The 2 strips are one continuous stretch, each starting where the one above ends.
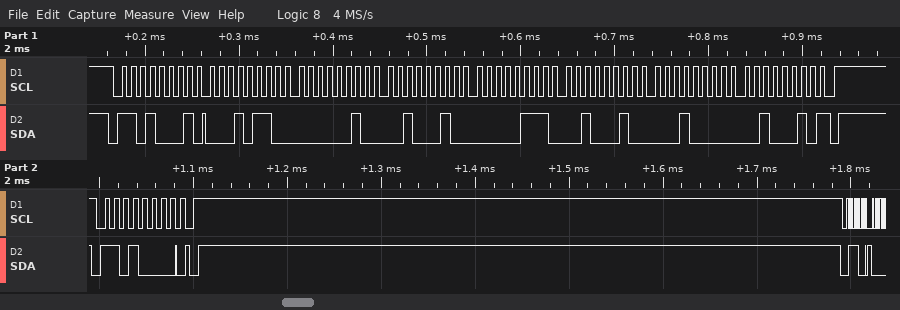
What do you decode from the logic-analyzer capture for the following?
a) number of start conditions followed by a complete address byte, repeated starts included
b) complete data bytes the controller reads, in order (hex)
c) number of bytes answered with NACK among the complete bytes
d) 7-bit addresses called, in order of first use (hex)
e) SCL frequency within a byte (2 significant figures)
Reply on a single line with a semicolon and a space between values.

2; 16 02 22 07 22 10 22; 1; 0x68; 100 kHz
